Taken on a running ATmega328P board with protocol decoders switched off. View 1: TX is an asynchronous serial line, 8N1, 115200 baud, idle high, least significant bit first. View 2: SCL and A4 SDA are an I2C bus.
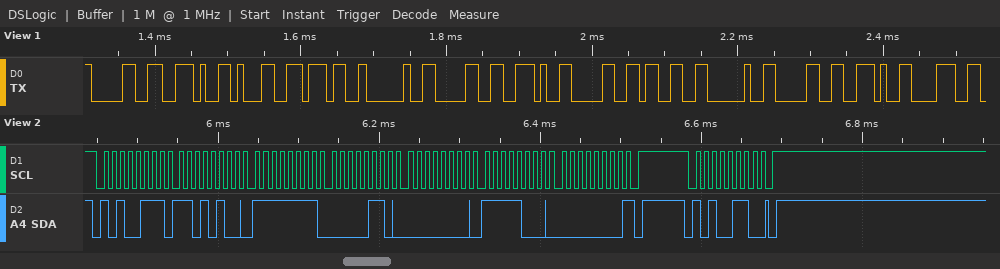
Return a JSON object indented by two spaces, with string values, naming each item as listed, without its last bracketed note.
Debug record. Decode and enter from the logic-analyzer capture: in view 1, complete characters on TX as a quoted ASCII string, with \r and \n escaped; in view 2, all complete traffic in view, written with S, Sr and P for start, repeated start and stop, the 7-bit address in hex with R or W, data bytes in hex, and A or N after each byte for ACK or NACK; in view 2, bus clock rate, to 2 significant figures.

{
  "in view 1, complete characters on TX as a quoted ASCII string, with \\r and \\n escaped": "\"0.17 0.03 0.8\"",
  "in view 2, all complete traffic in view, written with S, Sr and P for start, repeated start and stop, the 7-bit address in hex with R or W, data bytes in hex, and A or N after each byte for ACK or NACK": "S 53R A D4 A FF A 06 A 00 A F8 A 00 N P S 53W A P",
  "in view 2, bus clock rate, to 2 significant figures": "100 kHz"
}
